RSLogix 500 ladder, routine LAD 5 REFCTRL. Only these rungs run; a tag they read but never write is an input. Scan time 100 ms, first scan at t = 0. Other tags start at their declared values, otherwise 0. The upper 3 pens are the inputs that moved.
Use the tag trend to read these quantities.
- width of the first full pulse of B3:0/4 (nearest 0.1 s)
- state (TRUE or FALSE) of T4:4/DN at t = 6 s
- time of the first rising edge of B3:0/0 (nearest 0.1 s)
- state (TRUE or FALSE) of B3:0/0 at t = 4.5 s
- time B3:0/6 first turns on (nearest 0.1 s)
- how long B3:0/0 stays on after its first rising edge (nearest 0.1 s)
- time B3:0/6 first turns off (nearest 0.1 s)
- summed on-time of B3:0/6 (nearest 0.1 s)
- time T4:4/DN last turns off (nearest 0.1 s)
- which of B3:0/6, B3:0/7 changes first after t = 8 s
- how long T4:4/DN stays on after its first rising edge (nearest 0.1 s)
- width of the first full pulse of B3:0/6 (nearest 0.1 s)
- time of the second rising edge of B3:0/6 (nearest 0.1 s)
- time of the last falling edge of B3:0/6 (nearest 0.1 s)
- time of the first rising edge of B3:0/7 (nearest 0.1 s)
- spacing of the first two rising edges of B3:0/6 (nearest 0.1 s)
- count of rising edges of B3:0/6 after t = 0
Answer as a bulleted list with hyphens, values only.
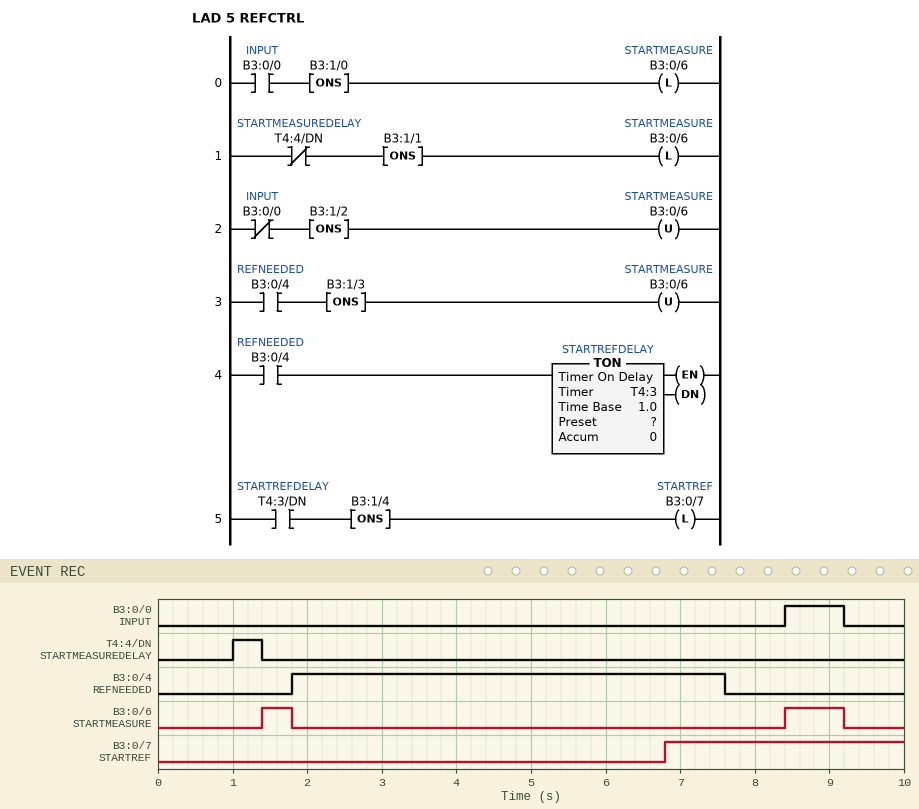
- 5.8 s
- FALSE
- 8.4 s
- FALSE
- 1.4 s
- 0.8 s
- 1.8 s
- 1.2 s
- 1.4 s
- B3:0/6
- 0.4 s
- 0.4 s
- 8.4 s
- 9.2 s
- 6.8 s
- 7.0 s
- 2
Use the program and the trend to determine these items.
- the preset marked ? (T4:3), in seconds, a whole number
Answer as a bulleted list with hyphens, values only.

- 5 s
